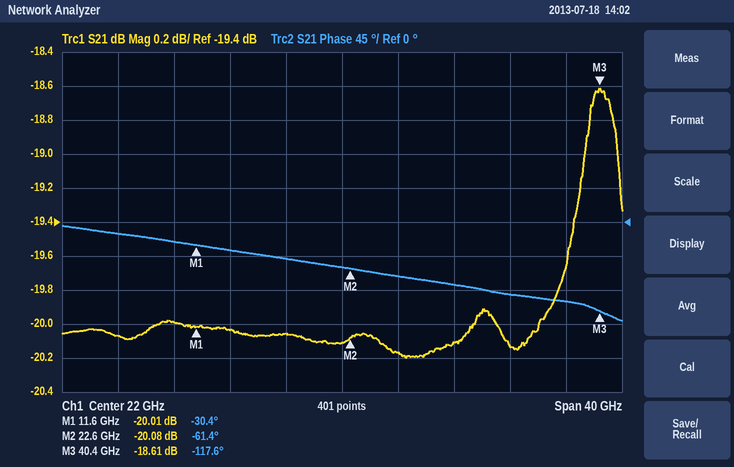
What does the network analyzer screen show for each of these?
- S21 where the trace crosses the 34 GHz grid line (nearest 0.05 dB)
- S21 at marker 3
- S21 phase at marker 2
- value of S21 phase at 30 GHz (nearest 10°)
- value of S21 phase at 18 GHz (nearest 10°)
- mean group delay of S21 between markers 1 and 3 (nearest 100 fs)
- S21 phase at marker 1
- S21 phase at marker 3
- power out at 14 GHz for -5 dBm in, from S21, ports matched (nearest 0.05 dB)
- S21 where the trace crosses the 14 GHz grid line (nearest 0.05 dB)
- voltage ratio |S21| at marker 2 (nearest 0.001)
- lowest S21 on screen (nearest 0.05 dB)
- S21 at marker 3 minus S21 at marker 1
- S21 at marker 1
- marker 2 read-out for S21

-20.15 dB
-18.61 dB
-61.4°
-80°
-50°
8.4 ps
-30.4°
-117.6°
-25.05 dBm
-20.05 dB
0.099
-20.20 dB
1.40 dB
-20.01 dB
-20.08 dB
